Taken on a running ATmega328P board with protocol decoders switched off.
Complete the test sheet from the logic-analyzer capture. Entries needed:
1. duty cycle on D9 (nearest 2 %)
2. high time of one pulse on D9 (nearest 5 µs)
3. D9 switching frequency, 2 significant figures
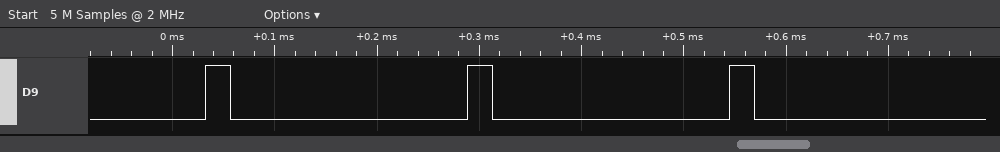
10 %
25 µs
3.9 kHz
